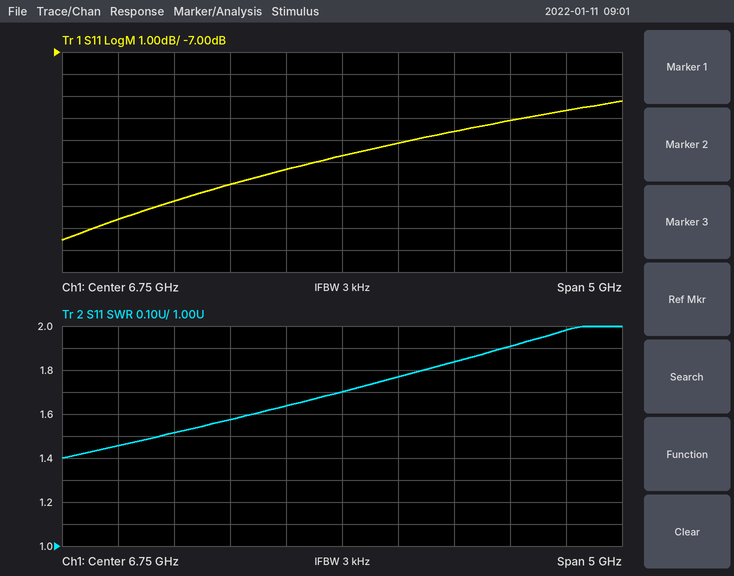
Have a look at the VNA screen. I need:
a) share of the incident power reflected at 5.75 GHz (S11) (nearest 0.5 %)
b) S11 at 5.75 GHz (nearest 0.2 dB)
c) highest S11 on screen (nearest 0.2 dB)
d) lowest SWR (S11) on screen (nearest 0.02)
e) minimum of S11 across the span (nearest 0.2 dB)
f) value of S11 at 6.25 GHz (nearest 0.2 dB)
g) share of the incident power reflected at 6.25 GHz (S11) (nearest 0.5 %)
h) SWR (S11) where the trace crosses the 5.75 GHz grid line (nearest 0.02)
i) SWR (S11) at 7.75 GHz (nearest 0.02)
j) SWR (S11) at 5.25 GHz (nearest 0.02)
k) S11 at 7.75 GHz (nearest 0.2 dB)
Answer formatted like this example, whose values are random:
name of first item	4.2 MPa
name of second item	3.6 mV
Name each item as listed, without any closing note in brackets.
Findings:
share of the incident power reflected at 5.75 GHz (S11)	5.0 %
S11 at 5.75 GHz	-13.0 dB
highest S11 on screen	-9.2 dB
lowest SWR (S11) on screen	1.40
minimum of S11 across the span	-15.6 dB
value of S11 at 6.25 GHz	-12.4 dB
share of the incident power reflected at 6.25 GHz (S11)	6.0 %
SWR (S11) where the trace crosses the 5.75 GHz grid line	1.58
SWR (S11) at 7.75 GHz	1.84
SWR (S11) at 5.25 GHz	1.52
S11 at 7.75 GHz	-10.6 dB
